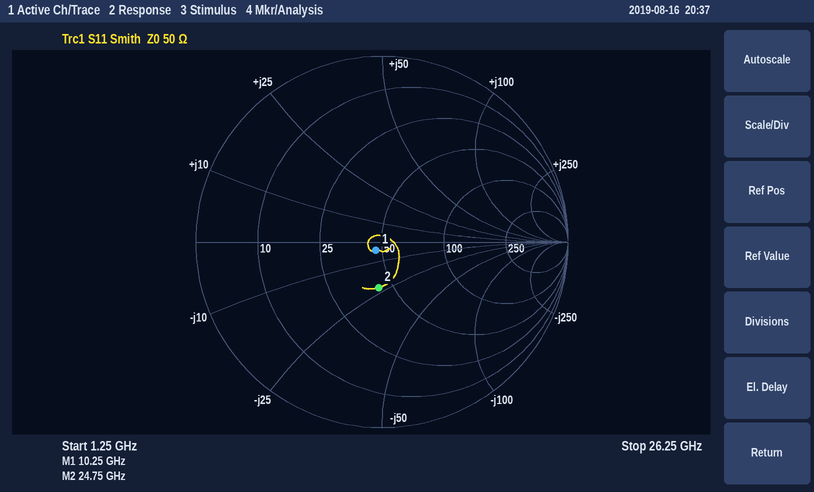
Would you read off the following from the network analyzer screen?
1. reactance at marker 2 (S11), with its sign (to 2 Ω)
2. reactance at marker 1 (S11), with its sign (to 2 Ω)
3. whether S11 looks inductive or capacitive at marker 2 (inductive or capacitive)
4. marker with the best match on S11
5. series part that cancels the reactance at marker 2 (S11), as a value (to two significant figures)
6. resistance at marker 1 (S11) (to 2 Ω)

-22 Ω
-4 Ω
capacitive
marker 1
140 pH
46 Ω
